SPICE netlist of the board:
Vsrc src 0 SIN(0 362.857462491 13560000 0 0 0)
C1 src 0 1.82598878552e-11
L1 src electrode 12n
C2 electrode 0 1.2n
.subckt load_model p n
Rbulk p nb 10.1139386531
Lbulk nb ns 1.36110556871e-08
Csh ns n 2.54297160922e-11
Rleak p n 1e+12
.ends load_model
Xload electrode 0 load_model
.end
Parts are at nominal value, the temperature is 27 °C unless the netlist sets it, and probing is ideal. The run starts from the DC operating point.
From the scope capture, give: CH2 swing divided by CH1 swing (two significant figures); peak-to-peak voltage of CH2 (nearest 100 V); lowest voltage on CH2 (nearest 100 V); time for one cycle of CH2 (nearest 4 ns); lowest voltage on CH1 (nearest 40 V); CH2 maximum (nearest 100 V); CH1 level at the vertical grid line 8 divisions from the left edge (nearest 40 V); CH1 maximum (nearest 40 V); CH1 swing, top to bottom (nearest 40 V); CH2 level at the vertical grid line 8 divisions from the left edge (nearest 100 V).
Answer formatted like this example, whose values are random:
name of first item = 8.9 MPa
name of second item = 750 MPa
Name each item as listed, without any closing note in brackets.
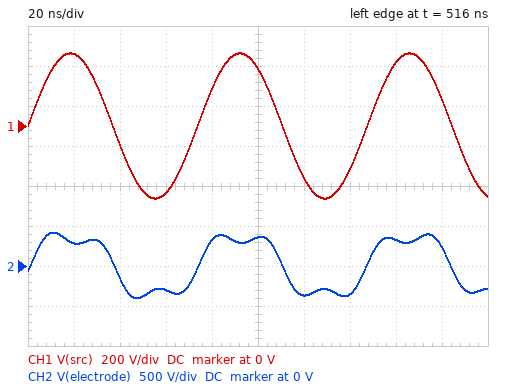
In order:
CH2 swing divided by CH1 swing = 1.1
peak-to-peak voltage of CH2 = 800 V
lowest voltage on CH2 = -400 V
time for one cycle of CH2 = 72 ns
lowest voltage on CH1 = -360 V
CH2 maximum = 400 V
CH1 level at the vertical grid line 8 divisions from the left edge = 320 V
CH1 maximum = 360 V
CH1 swing, top to bottom = 720 V
CH2 level at the vertical grid line 8 divisions from the left edge = 300 V
